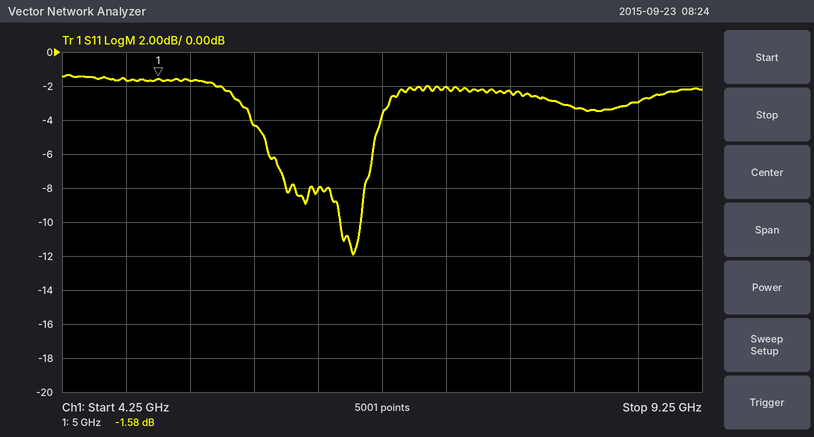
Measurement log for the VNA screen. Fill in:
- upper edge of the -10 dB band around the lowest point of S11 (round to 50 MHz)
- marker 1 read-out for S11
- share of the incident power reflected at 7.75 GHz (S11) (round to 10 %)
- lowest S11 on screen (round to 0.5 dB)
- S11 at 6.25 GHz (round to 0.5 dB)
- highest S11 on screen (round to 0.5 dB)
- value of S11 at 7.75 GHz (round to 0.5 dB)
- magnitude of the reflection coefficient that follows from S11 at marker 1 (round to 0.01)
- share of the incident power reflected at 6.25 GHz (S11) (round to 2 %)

6.60 GHz
-1.58 dB
60 %
-12.0 dB
-8.0 dB
-1.5 dB
-2.5 dB
0.83
16 %
